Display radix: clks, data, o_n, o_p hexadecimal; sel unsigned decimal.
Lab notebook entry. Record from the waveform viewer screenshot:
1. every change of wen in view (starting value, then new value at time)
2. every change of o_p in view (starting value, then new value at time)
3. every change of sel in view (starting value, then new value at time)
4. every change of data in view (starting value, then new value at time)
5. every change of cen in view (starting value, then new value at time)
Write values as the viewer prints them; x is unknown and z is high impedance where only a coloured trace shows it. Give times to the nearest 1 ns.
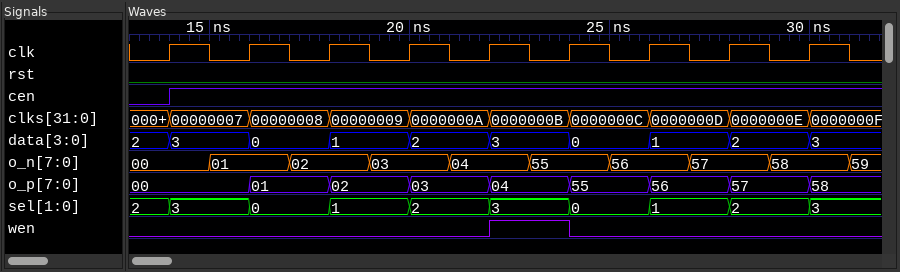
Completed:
0, 1 at 22 ns, 0 at 24 ns
00, 01 at 16 ns, 02 at 18 ns, 03 at 20 ns, 04 at 22 ns, 55 at 24 ns, 56 at 26 ns, 57 at 28 ns, 58 at 30 ns
2, 3 at 14 ns, 0 at 16 ns, 1 at 18 ns, 2 at 20 ns, 3 at 22 ns, 0 at 24 ns, 1 at 26 ns, 2 at 28 ns, 3 at 30 ns
2, 3 at 14 ns, 0 at 16 ns, 1 at 18 ns, 2 at 20 ns, 3 at 22 ns, 0 at 24 ns, 1 at 26 ns, 2 at 28 ns, 3 at 30 ns
0, 1 at 14 ns
